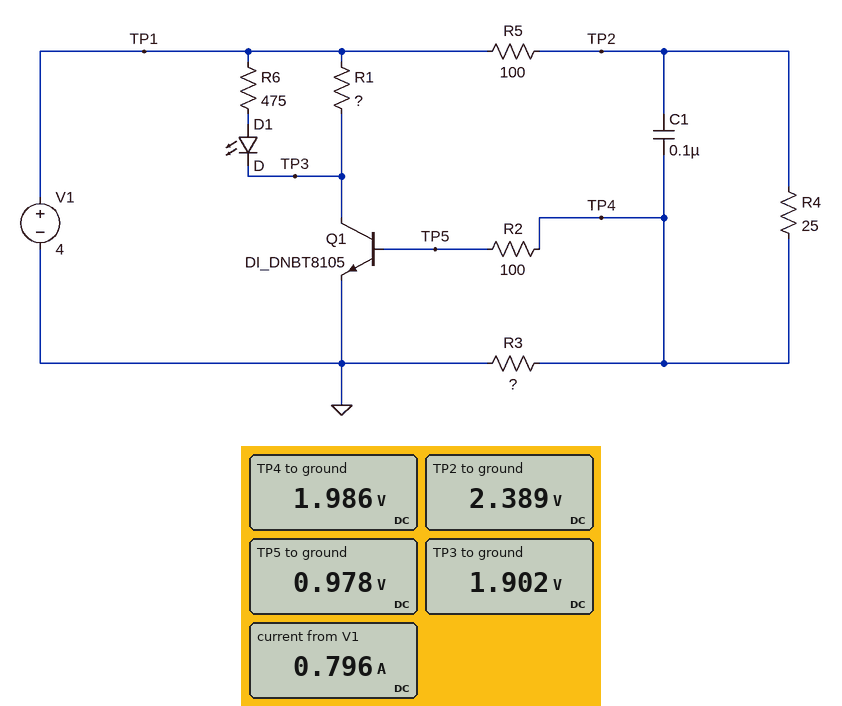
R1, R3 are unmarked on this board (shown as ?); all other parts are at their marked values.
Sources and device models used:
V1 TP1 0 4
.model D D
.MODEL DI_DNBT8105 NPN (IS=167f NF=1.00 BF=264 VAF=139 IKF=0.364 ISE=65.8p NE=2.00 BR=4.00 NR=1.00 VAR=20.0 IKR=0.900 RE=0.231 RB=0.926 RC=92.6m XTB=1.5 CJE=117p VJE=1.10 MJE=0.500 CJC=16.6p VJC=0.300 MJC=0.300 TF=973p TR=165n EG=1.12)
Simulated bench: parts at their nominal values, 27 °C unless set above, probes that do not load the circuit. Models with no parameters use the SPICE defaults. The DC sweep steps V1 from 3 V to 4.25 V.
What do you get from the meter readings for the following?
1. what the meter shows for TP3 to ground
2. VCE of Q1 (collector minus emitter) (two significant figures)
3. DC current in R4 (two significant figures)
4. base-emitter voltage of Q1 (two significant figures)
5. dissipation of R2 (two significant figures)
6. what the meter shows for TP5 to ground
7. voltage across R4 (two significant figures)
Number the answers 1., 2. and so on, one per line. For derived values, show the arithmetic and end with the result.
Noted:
1. 1.902 V
2. 1.902 V = 1.9 V
3. (2.389 V - 1.986 V) / 25 Ω = 16 mA
4. 978 mV = 980 mV
5. (1.986 V - 978 mV)^2 / 100 Ω = 10 mW
6. 0.978 V
7. 2.389 V - 1.986 V = 400 mV
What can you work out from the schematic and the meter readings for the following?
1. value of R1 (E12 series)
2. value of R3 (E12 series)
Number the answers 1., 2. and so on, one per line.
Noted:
1. 2.7 Ω
2. 330 Ω
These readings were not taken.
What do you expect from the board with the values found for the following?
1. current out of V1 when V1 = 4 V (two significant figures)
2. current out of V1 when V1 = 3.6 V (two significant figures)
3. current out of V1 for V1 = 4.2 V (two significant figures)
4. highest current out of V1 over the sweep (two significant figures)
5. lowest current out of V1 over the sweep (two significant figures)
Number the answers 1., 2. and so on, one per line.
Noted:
1. 800 mA
2. 730 mA
3. 830 mA
4. 840 mA
5. 610 mA
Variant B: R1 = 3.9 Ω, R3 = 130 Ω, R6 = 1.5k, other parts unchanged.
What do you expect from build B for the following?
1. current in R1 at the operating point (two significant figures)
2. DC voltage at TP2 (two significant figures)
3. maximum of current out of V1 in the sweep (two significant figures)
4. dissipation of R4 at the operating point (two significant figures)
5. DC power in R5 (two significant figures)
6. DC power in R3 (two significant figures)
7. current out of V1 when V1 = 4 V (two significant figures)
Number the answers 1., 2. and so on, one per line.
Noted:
1. 610 mA
2. 2.1 V
3. 670 mA
4. 9.2 mW
5. 37 mW
6. 20 mW
7. 630 mA
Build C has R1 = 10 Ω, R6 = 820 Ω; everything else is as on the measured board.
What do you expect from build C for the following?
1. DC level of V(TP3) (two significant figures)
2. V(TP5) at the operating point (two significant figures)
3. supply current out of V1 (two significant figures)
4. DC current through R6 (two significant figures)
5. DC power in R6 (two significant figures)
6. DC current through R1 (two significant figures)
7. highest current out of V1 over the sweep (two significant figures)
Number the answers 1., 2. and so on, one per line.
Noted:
1. 220 mV
2. 860 mV
3. 400 mA
4. 3.8 mA
5. 12 mW
6. 380 mA
7. 420 mA
